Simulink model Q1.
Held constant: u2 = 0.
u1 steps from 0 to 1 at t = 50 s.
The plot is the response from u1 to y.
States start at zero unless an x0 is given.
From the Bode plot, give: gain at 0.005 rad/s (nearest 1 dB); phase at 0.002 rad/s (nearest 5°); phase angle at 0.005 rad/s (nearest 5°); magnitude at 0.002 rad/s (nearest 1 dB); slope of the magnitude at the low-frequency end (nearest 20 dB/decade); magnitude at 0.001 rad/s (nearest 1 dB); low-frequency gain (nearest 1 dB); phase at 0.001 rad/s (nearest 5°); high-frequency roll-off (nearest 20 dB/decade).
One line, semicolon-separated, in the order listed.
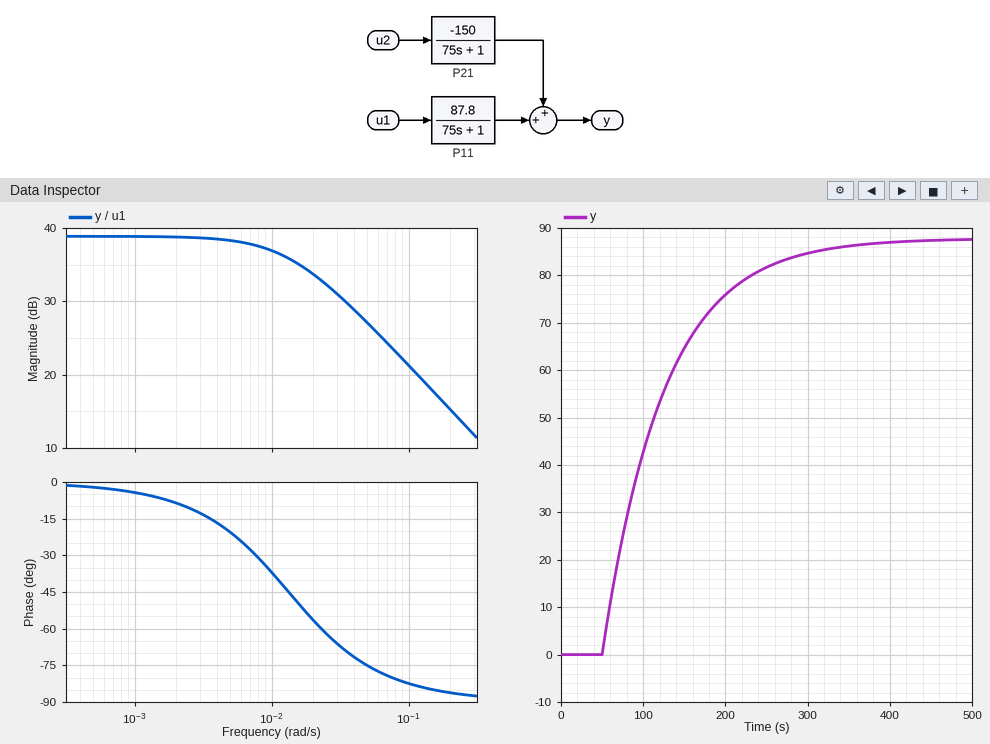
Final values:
38 dB; -10°; -20°; 39 dB; 0 dB/decade; 39 dB; 39 dB; -5°; -20 dB/decade
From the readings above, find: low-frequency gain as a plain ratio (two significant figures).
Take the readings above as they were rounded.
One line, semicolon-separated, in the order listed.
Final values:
89
